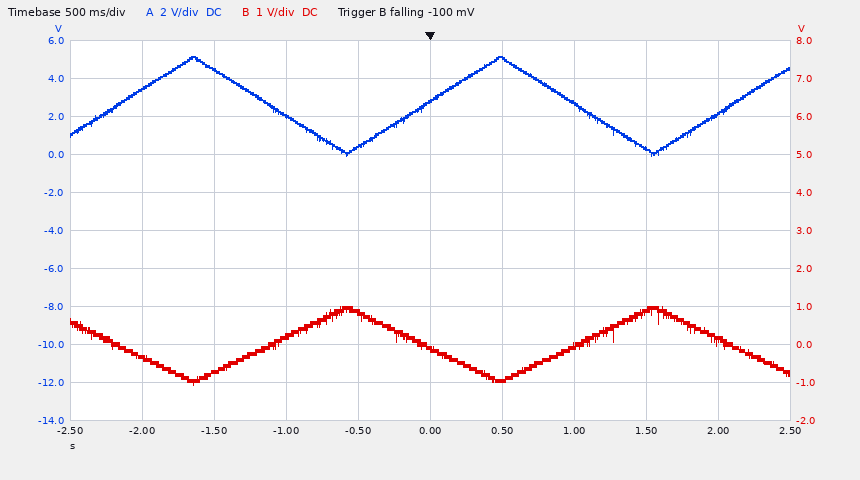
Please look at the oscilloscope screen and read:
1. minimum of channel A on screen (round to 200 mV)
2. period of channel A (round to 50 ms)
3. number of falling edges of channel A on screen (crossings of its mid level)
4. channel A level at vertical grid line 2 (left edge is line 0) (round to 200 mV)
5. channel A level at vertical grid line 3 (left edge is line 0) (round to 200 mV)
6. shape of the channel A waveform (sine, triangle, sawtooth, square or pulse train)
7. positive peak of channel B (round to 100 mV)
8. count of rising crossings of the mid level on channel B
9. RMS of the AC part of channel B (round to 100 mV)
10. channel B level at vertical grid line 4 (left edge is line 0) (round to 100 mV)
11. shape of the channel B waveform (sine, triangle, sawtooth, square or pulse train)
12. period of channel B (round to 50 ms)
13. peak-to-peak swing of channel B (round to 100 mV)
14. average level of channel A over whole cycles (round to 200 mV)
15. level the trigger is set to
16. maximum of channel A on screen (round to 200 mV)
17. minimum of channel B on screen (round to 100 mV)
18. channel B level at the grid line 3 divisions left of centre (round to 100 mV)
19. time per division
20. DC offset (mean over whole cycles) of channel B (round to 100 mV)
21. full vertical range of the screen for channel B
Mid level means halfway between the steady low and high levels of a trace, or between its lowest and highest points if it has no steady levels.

-200 mV
2.15 s
2
4.4 V
2.0 V
triangle
1.0 V
2
600 mV
800 mV
triangle
2.15 s
2.1 V
2.6 V
-100 mV
5.2 V
-1.1 V
-700 mV
500 ms
0.0 V
10 V
